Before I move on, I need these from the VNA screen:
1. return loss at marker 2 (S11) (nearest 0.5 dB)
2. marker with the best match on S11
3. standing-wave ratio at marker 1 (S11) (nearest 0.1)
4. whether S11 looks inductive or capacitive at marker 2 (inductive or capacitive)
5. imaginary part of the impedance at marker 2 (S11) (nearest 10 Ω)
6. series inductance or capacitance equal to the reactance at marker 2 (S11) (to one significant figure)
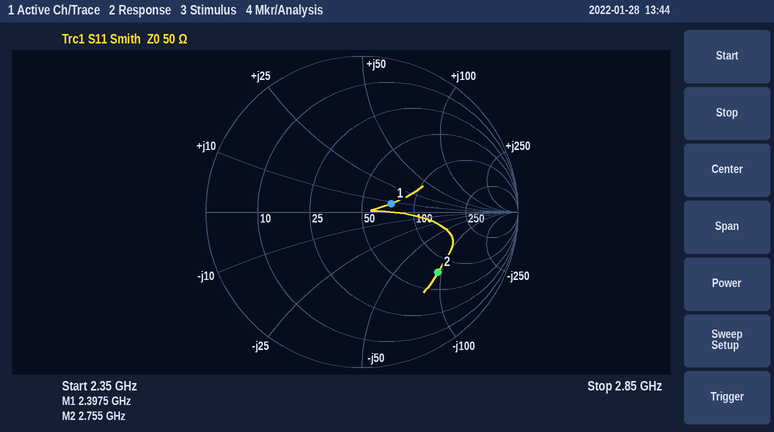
4.0 dB
marker 1
1.5
capacitive
-90 Ω
600 fF
